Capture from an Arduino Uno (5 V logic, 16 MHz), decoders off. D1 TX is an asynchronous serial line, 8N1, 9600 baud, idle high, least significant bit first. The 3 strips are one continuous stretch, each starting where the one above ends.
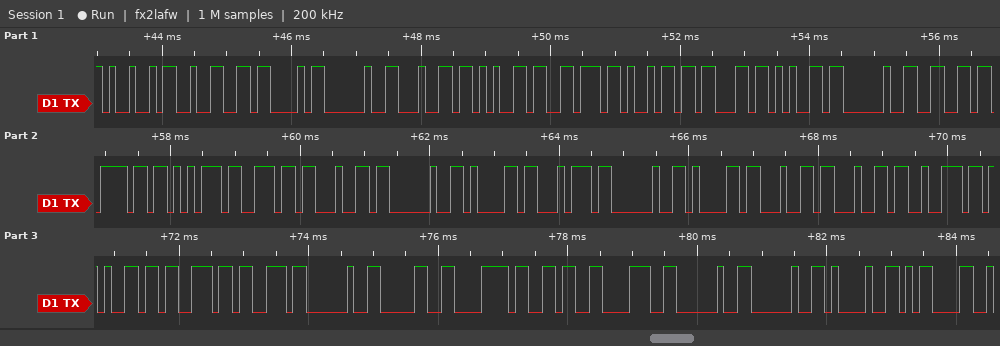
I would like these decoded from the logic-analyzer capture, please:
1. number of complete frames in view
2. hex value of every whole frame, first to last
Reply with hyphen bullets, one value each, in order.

- 36
- 49 32 43 20 64 65 76 69 63 65 20 66 6F 75 6E 64 20 61 74 20 61 64 64 72 65 73 73 20 30 78 36 38 20 20 21 0D
